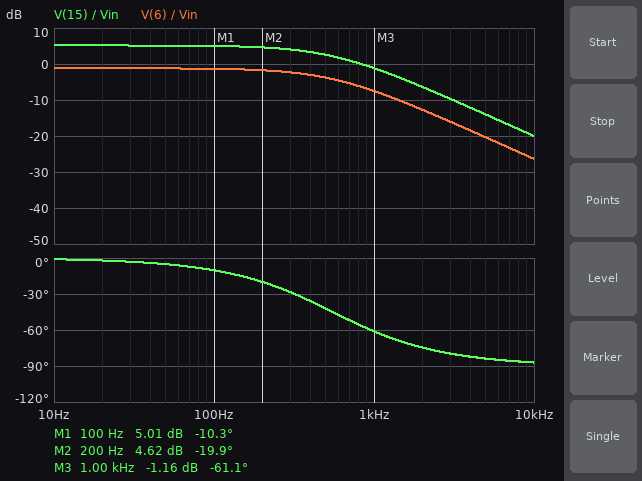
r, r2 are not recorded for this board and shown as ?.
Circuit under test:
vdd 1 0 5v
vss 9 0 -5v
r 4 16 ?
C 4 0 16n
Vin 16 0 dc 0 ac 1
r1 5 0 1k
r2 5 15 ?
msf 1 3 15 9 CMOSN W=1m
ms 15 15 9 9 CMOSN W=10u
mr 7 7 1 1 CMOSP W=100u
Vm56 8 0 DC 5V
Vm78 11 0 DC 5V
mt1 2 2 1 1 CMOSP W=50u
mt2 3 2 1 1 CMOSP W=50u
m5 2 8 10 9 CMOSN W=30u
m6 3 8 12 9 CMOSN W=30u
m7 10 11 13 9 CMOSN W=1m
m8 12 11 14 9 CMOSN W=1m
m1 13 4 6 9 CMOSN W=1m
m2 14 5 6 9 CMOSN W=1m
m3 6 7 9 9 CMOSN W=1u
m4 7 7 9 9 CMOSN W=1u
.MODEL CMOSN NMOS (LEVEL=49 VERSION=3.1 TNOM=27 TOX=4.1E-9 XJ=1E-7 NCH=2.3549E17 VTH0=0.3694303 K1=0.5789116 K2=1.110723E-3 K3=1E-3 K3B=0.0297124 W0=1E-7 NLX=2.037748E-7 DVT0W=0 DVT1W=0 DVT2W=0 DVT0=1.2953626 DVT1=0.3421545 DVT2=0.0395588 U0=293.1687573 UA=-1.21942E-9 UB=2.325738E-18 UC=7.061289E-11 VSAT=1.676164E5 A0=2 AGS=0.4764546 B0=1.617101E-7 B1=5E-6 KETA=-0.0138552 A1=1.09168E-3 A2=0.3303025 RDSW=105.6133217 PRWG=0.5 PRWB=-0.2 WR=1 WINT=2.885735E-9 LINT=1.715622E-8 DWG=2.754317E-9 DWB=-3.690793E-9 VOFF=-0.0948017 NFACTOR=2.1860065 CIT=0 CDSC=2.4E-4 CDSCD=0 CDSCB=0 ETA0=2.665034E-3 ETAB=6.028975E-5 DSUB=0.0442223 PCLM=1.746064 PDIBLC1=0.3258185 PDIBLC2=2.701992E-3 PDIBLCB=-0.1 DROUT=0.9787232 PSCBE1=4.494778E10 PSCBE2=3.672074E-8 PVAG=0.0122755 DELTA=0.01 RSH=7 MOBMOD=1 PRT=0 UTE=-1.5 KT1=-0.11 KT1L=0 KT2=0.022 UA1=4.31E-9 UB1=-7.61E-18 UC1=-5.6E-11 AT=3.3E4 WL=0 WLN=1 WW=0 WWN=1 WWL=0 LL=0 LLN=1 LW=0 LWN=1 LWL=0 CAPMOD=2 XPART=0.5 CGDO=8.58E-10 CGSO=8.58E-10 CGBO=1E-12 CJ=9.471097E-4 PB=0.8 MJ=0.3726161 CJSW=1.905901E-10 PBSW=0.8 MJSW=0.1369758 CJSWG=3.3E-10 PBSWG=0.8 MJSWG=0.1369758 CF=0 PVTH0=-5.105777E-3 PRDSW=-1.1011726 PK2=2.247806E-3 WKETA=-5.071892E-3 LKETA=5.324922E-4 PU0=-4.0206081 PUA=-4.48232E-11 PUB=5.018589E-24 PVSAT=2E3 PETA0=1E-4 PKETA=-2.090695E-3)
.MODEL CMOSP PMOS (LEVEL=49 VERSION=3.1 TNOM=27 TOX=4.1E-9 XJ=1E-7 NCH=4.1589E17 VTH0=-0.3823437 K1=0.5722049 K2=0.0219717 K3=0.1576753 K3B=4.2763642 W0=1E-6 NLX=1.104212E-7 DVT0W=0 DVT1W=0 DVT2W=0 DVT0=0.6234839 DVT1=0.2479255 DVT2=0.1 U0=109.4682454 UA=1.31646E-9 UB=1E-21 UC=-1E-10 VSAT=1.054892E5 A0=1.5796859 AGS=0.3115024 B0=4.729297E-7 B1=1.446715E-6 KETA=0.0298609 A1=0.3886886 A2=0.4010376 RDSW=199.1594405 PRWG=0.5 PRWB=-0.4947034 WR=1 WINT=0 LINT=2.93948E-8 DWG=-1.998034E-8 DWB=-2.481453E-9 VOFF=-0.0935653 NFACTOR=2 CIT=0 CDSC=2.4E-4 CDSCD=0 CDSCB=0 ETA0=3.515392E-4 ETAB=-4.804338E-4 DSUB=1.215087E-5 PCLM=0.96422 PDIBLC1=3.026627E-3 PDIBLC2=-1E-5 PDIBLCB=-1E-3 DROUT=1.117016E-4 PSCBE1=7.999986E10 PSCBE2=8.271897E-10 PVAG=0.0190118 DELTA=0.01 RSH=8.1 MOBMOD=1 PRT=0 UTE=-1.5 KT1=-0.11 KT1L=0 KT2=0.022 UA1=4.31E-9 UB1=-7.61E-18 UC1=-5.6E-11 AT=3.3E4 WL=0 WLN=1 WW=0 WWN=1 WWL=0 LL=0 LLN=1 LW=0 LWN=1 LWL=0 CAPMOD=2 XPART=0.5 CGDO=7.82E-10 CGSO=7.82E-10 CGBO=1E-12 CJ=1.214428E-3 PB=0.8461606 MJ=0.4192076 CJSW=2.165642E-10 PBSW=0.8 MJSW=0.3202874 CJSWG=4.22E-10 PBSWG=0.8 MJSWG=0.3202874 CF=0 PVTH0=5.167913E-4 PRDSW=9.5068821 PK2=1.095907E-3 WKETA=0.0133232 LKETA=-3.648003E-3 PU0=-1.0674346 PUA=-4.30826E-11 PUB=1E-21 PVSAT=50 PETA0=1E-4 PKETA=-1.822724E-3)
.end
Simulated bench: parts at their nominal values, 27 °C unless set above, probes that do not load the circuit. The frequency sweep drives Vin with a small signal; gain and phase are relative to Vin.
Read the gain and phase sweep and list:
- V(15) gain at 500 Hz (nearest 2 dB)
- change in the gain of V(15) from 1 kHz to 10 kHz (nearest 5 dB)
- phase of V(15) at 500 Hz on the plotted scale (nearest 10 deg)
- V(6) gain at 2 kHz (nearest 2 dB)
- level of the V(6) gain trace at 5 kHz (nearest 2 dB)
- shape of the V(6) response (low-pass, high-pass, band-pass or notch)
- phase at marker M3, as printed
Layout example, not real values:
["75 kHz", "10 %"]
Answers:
["2 dB", "-20 dB", "-40 deg", "-12 dB", "-20 dB", "low-pass", "-61.1 deg"]
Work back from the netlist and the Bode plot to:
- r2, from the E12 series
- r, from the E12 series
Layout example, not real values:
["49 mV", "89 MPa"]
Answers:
["820 Ω", "18 kΩ"]
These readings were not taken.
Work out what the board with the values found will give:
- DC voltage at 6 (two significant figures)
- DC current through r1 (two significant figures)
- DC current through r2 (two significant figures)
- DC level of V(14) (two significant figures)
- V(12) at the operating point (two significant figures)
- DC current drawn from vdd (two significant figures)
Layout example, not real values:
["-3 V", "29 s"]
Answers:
["-1.1 V", "4.7 µA", "4.7 µA", "1.5 V", "1.5 V", "3.0 mA"]
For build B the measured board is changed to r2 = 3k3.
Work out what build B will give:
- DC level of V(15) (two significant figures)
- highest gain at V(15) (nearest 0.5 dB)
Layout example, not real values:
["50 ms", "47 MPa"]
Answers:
["20 mV", "12.5 dB"]
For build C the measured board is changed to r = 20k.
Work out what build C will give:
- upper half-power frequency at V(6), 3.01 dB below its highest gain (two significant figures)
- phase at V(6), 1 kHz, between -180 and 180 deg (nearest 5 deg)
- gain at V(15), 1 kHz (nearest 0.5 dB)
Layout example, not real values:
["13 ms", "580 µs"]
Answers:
["500 Hz", "-65 deg", "-2.0 dB"]
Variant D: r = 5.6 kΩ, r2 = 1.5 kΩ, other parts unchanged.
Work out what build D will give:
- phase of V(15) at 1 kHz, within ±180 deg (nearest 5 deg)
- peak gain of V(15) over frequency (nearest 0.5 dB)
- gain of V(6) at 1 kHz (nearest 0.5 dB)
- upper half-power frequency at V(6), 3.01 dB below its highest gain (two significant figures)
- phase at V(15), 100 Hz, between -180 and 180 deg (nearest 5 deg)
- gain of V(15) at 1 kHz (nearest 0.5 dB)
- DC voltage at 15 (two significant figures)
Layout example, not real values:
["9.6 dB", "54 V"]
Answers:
["-30 deg", "8.0 dB", "-2.5 dB", "1.8 kHz", "-5 deg", "6.5 dB", "12 mV"]
